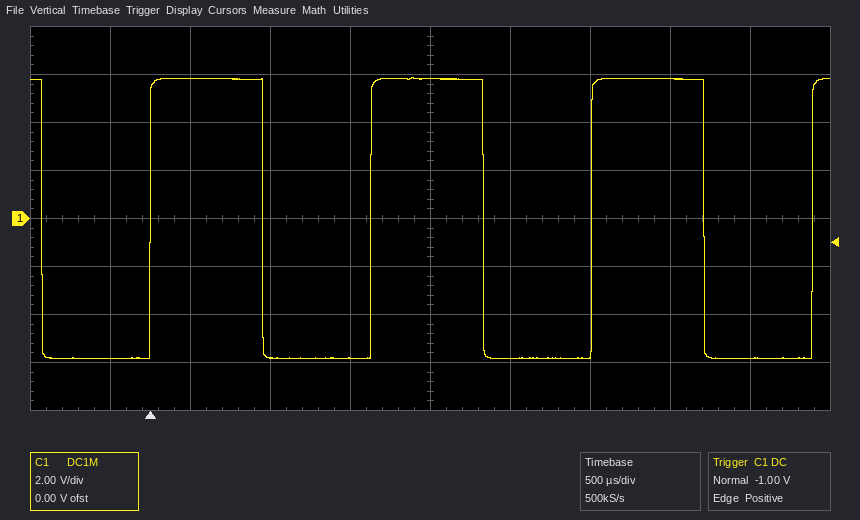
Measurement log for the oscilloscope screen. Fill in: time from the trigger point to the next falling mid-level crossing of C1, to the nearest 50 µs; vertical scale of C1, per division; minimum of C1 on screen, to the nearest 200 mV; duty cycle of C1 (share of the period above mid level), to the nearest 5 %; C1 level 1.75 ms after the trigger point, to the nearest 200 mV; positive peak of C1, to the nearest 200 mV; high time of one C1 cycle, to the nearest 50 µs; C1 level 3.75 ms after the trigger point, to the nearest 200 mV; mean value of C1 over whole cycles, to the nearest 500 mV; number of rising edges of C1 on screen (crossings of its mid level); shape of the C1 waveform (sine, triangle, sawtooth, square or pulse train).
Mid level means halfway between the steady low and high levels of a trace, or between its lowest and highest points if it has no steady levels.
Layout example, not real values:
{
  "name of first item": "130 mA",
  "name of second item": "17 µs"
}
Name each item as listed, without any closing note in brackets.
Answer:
{
  "time from the trigger point to the next falling mid-level crossing of C1, to the nearest 50 µs": "700 µs",
  "vertical scale of C1, per division": "2 V",
  "minimum of C1 on screen, to the nearest 200 mV": "-5.8 V",
  "duty cycle of C1 (share of the period above mid level), to the nearest 5 %": "50 %",
  "C1 level 1.75 ms after the trigger point, to the nearest 200 mV": "5.8 V",
  "positive peak of C1, to the nearest 200 mV": "5.8 V",
  "high time of one C1 cycle, to the nearest 50 µs": "700 µs",
  "C1 level 3.75 ms after the trigger point, to the nearest 200 mV": "-5.8 V",
  "mean value of C1 over whole cycles, to the nearest 500 mV": "0.0 V",
  "number of rising edges of C1 on screen": "4",
  "shape of the C1 waveform": "square"
}
